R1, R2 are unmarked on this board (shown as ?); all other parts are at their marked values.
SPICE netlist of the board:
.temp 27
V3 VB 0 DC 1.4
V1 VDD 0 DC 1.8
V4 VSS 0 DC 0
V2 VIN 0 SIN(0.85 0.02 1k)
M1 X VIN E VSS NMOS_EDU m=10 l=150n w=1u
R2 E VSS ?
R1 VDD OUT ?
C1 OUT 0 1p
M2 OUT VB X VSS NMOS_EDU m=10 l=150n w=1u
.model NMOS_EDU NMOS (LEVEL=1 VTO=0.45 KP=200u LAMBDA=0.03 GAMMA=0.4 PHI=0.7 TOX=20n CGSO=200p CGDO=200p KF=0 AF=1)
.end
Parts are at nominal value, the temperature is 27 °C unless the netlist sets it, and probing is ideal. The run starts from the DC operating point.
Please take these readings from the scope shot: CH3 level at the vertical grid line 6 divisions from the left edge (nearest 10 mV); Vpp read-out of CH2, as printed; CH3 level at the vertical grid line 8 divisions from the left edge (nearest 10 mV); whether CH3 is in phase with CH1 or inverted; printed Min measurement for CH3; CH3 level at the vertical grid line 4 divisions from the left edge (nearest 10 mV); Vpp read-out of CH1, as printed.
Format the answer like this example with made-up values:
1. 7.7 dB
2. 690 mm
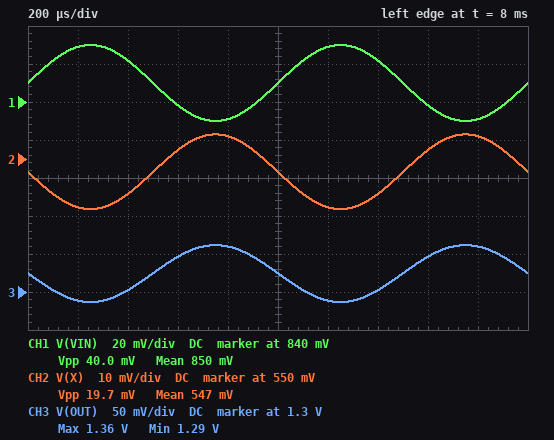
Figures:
1. 1.29 V
2. 19.7 mV
3. 1.35 V
4. inverted
5. 1.29 V
6. 1.36 V
7. 40.0 mV
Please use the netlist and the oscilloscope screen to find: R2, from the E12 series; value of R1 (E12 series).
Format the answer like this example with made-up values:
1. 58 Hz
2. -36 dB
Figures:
1. 150 Ω
2. 820 Ω
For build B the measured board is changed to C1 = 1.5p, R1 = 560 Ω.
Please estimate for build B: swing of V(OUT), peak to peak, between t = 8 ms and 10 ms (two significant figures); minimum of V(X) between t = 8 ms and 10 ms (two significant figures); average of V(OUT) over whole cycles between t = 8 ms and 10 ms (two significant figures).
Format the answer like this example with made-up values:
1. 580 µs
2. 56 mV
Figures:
1. 51 mV
2. 540 mV
3. 1.5 V
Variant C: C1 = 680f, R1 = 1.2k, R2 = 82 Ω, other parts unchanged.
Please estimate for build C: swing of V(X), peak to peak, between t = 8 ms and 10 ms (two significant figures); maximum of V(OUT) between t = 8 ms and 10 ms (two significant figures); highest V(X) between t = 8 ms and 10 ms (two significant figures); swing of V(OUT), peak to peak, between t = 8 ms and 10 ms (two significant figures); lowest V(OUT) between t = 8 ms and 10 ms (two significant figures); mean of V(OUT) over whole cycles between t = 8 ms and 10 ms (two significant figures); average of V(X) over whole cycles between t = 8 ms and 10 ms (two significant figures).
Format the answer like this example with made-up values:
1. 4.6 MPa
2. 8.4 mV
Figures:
1. 24 mV
2. 1.0 V
3. 530 mV
4. 150 mV
5. 860 mV
6. 930 mV
7. 520 mV
